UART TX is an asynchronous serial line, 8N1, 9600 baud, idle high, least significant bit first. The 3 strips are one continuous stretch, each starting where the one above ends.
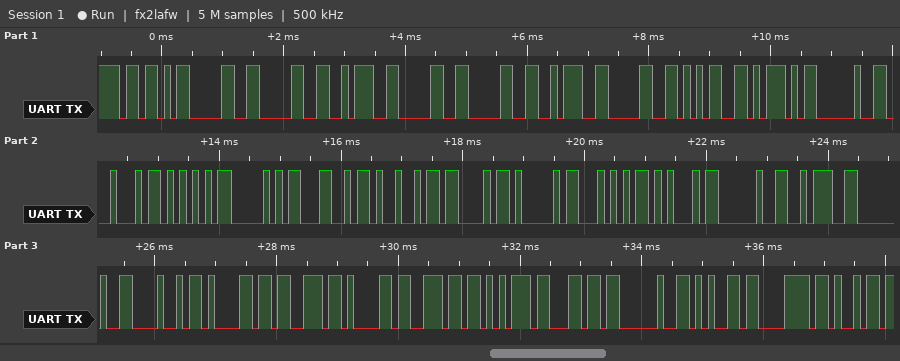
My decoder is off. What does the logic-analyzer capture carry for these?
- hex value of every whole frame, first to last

5B 30 30 3A 30 30 3A 30 35 5D 20 44 55 50 4C 49 43 41 54 45 20 3A 20 48 61 73 61 6E 75 6C 20 65 78 69
